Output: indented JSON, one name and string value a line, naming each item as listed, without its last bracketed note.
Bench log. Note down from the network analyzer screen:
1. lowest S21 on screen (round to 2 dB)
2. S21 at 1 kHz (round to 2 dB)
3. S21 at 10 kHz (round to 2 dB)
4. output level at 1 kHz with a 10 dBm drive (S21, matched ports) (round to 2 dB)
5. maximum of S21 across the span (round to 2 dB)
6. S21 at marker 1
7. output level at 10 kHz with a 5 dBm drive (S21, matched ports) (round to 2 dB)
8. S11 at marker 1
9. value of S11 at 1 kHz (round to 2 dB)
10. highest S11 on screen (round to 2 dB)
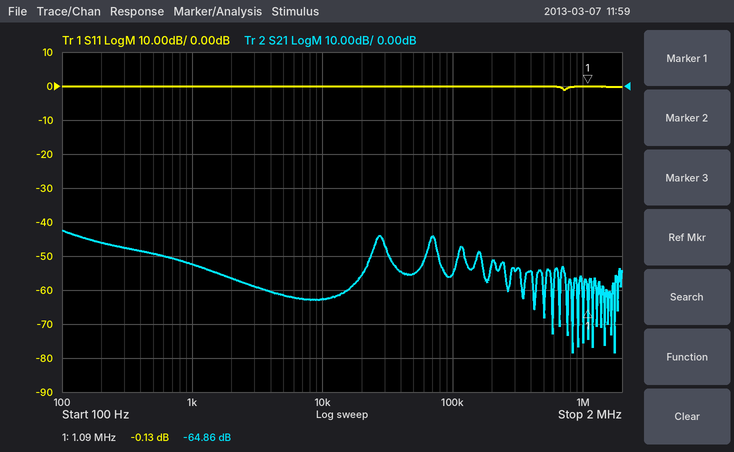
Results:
{
  "lowest S21 on screen": "-78 dB",
  "S21 at 1 kHz": "-52 dB",
  "S21 at 10 kHz": "-62 dB",
  "output level at 1 kHz with a 10 dBm drive (S21, matched ports)": "-42 dBm",
  "maximum of S21 across the span": "-42 dB",
  "S21 at marker 1": "-64.86 dB",
  "output level at 10 kHz with a 5 dBm drive (S21, matched ports)": "-58 dBm",
  "S11 at marker 1": "-0.13 dB",
  "value of S11 at 1 kHz": "0 dB",
  "highest S11 on screen": "0 dB"
}
